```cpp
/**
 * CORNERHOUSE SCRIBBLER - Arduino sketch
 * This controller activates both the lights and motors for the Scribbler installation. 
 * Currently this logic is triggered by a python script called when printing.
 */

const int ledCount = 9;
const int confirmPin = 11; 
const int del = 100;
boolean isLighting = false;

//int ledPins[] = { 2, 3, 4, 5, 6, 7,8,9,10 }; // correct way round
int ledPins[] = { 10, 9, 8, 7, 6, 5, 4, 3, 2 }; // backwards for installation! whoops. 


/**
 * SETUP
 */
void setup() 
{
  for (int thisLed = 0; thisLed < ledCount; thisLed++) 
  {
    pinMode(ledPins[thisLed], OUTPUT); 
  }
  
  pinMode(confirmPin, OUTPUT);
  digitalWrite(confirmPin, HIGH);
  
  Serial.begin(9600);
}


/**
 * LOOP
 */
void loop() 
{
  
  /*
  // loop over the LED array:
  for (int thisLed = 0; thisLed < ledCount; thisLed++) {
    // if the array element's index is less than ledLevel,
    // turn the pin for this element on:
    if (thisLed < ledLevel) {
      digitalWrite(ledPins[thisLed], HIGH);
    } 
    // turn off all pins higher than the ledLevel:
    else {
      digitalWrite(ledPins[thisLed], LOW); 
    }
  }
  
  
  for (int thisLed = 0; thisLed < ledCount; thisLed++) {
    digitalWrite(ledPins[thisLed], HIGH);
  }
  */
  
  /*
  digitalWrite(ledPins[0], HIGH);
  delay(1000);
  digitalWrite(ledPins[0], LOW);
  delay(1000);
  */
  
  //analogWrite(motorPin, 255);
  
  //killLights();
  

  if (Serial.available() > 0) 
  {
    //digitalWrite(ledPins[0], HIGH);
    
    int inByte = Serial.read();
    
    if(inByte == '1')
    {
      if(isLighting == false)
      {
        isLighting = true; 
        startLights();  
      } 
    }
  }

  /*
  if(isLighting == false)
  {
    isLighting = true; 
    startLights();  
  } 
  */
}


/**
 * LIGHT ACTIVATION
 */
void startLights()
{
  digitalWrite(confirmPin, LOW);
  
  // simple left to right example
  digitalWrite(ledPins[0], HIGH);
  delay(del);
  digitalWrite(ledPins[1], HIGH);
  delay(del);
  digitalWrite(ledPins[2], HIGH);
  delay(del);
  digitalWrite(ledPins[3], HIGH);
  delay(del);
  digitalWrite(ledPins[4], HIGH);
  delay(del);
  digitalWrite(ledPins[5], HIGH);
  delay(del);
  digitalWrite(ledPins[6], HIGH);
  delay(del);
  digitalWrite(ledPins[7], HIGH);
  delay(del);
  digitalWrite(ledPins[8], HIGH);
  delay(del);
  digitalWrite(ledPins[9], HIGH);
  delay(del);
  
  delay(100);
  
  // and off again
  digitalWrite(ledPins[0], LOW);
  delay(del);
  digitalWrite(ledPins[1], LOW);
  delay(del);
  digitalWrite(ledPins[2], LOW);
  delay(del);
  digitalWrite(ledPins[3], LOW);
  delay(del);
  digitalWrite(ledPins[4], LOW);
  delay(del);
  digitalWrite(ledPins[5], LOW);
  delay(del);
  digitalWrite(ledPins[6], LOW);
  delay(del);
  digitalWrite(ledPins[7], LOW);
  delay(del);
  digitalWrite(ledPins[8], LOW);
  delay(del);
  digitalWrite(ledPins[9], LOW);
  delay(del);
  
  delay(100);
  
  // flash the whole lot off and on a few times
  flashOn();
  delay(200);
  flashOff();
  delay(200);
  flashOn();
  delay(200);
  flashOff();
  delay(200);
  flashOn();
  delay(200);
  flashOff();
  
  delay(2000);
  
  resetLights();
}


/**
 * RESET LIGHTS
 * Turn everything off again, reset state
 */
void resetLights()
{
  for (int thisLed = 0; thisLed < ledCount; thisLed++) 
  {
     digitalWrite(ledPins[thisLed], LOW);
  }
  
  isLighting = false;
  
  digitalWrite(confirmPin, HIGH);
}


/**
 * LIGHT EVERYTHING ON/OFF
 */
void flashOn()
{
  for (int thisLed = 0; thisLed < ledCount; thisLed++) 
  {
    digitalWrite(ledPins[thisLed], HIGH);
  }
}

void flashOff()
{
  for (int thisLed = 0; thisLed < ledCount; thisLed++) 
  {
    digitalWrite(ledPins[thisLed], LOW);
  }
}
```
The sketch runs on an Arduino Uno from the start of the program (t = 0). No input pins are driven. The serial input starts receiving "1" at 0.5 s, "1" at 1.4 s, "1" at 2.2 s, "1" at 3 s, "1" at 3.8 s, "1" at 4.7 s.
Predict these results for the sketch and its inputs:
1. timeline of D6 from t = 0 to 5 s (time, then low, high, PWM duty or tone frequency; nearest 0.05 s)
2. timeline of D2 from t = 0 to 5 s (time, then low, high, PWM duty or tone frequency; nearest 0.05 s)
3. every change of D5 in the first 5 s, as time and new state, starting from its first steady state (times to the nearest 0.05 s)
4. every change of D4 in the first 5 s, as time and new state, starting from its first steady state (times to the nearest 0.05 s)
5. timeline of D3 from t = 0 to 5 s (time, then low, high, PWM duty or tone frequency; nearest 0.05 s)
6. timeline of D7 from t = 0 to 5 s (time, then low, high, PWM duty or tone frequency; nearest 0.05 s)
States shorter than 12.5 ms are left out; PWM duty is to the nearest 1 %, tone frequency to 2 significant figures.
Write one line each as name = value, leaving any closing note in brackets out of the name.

timeline of D6 from t = 0 to 5 s = 0 s low; 0.9 s high; 2 s low; 2.7 s high; 2.9 s low; 3.1 s high; 3.3 s low; 3.5 s high; 3.7 s low
timeline of D2 from t = 0 to 5 s = 0 s low; 1.3 s high; 2.4 s low; 2.7 s high; 2.9 s low; 3.1 s high; 3.3 s low; 3.5 s high; 3.7 s low
every change of D5 in the first 5 s, as time and new state, starting from its first steady state = 0 s low; 1 s high; 2.1 s low; 2.7 s high; 2.9 s low; 3.1 s high; 3.3 s low; 3.5 s high; 3.7 s low
every change of D4 in the first 5 s, as time and new state, starting from its first steady state = 0 s low; 1.1 s high; 2.2 s low; 2.7 s high; 2.9 s low; 3.1 s high; 3.3 s low; 3.5 s high; 3.7 s low
timeline of D3 from t = 0 to 5 s = 0 s low; 1.2 s high; 2.3 s low; 2.7 s high; 2.9 s low; 3.1 s high; 3.3 s low; 3.5 s high; 3.7 s low
timeline of D7 from t = 0 to 5 s = 0 s low; 0.8 s high; 1.9 s low; 2.7 s high; 2.9 s low; 3.1 s high; 3.3 s low; 3.5 s high; 3.7 s low
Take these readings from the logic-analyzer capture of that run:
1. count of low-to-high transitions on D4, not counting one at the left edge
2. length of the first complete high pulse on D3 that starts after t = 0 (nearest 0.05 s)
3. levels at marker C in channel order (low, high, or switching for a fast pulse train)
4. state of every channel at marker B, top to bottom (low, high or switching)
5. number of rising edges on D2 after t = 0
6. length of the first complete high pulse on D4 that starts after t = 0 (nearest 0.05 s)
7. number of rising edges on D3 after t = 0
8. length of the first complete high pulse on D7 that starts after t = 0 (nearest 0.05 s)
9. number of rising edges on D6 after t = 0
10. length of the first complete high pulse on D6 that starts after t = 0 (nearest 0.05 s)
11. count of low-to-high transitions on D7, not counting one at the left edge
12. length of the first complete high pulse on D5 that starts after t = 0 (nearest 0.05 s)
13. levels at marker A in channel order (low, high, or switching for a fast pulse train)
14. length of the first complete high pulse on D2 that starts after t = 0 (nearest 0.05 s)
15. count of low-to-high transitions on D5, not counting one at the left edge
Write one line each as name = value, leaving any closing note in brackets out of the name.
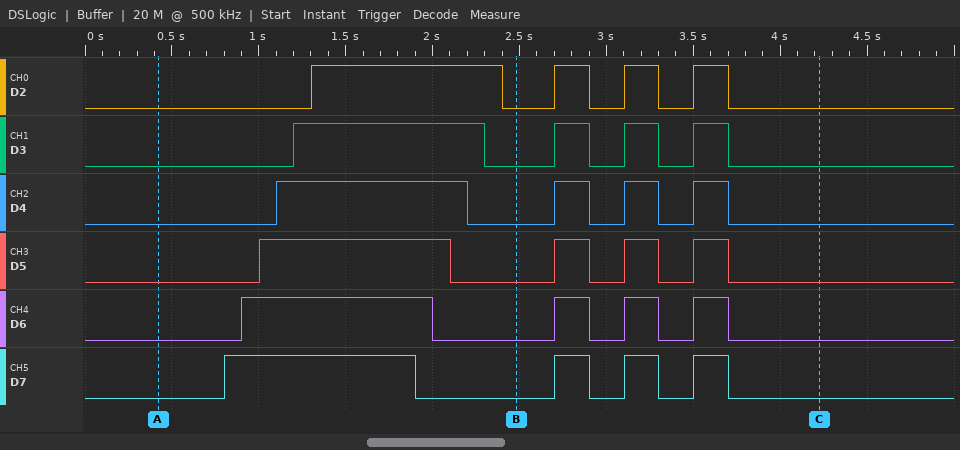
count of low-to-high transitions on D4, not counting one at the left edge = 4
length of the first complete high pulse on D3 that starts after t = 0 = 1.10 s
levels at marker C in channel order = D2 low, D3 low, D4 low, D5 low, D6 low, D7 low
state of every channel at marker B, top to bottom = D2 low, D3 low, D4 low, D5 low, D6 low, D7 low
number of rising edges on D2 after t = 0 = 4
length of the first complete high pulse on D4 that starts after t = 0 = 1.10 s
number of rising edges on D3 after t = 0 = 4
length of the first complete high pulse on D7 that starts after t = 0 = 1.10 s
number of rising edges on D6 after t = 0 = 4
length of the first complete high pulse on D6 that starts after t = 0 = 1.10 s
count of low-to-high transitions on D7, not counting one at the left edge = 4
length of the first complete high pulse on D5 that starts after t = 0 = 1.10 s
levels at marker A in channel order = D2 low, D3 low, D4 low, D5 low, D6 low, D7 low
length of the first complete high pulse on D2 that starts after t = 0 = 1.10 s
count of low-to-high transitions on D5, not counting one at the left edge = 4
